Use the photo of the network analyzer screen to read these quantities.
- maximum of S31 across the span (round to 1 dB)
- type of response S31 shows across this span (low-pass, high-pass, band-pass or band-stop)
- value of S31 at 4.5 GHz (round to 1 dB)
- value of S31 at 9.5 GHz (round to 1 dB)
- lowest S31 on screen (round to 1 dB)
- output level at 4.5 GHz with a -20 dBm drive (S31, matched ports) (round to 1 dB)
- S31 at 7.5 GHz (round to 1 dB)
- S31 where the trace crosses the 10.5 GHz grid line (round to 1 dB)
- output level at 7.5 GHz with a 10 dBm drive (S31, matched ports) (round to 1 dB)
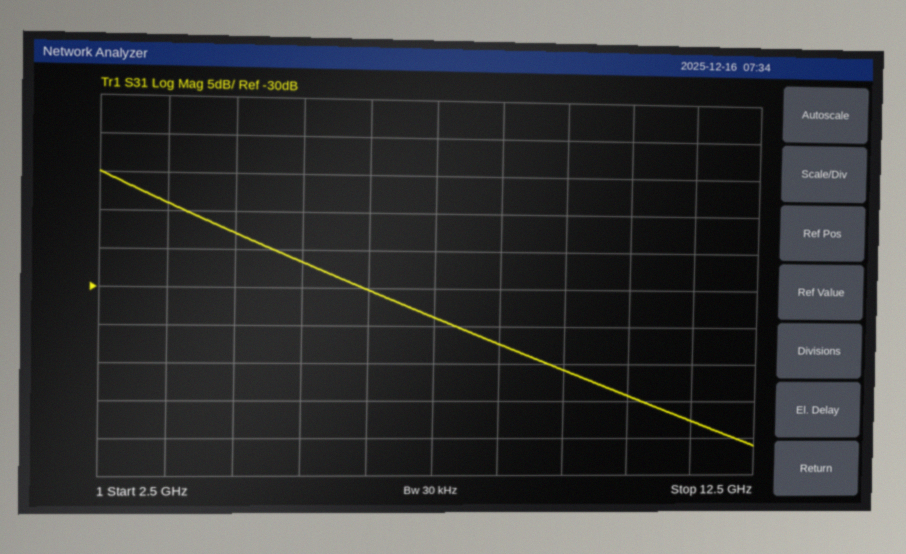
-15 dB
low-pass
-23 dB
-41 dB
-51 dB
-43 dBm
-34 dB
-44 dB
-24 dBm
